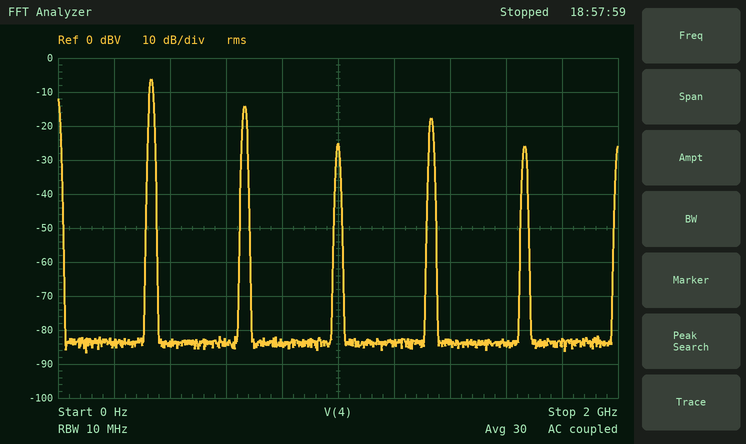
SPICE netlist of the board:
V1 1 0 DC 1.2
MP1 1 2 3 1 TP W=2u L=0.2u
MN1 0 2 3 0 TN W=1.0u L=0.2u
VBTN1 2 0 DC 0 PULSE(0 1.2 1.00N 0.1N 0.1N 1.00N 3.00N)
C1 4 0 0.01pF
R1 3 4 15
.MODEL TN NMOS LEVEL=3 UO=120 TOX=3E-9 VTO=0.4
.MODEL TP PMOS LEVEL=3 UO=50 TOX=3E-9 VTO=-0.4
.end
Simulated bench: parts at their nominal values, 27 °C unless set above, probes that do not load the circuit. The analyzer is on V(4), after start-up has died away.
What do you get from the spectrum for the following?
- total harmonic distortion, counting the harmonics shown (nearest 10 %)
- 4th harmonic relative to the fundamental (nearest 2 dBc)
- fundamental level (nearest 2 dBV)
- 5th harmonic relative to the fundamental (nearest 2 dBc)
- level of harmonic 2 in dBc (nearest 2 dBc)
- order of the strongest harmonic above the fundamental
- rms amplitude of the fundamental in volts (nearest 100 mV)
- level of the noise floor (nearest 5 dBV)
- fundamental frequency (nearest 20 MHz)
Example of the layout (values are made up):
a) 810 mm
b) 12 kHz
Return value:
a) 50 %
b) -12 dBc
c) -6 dBV
d) -20 dBc
e) -8 dBc
f) 2
g) 500 mV
h) -85 dBV
i) 340 MHz
